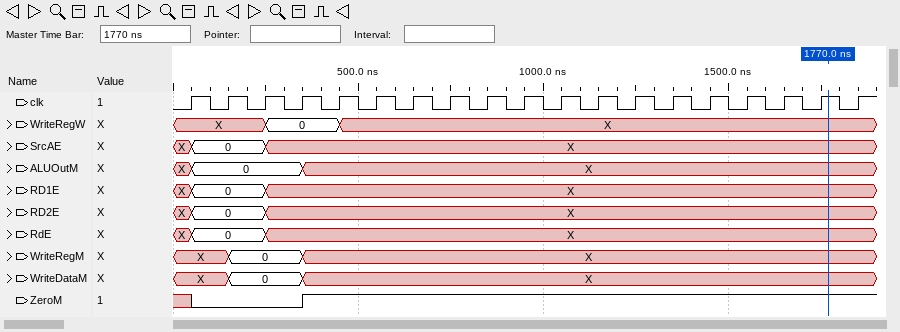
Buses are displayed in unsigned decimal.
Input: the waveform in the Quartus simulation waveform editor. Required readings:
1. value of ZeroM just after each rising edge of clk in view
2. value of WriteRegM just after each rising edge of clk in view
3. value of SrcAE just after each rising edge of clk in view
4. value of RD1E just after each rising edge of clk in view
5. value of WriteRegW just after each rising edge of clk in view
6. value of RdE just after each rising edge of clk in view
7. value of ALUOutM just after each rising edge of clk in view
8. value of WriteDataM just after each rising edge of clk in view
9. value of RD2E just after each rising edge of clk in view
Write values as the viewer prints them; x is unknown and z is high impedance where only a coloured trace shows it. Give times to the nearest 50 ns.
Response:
0 0 0 1 1 1 1 1 1 1 1 1 1 1 1 1 1 1 1
X, 0, 0, X, X, X, X, X, X, X, X, X, X, X, X, X, X, X, X
0, 0, X, X, X, X, X, X, X, X, X, X, X, X, X, X, X, X, X
0, 0, X, X, X, X, X, X, X, X, X, X, X, X, X, X, X, X, X
X, X, 0, 0, X, X, X, X, X, X, X, X, X, X, X, X, X, X, X
0, 0, X, X, X, X, X, X, X, X, X, X, X, X, X, X, X, X, X
0, 0, 0, X, X, X, X, X, X, X, X, X, X, X, X, X, X, X, X
X, 0, 0, X, X, X, X, X, X, X, X, X, X, X, X, X, X, X, X
0, 0, X, X, X, X, X, X, X, X, X, X, X, X, X, X, X, X, X
